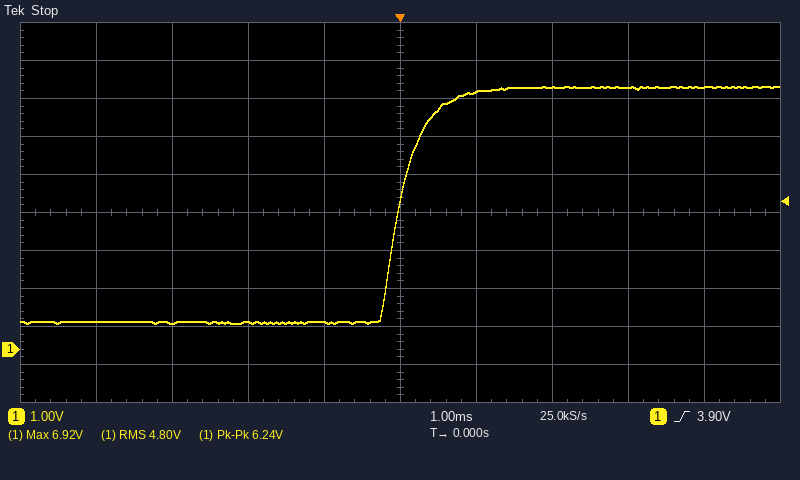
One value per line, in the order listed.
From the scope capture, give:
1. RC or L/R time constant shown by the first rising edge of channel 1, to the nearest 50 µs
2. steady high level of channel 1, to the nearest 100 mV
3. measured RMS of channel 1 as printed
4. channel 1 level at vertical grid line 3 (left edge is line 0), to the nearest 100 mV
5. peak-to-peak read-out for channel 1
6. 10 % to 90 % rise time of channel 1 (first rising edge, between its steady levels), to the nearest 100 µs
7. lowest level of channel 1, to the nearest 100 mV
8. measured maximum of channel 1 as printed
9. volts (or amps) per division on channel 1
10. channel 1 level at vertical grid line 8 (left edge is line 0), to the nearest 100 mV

300 µs
6.9 V
4.80 V
700 mV
6.24 V
700 µs
700 mV
6.92 V
1 V
6.9 V
